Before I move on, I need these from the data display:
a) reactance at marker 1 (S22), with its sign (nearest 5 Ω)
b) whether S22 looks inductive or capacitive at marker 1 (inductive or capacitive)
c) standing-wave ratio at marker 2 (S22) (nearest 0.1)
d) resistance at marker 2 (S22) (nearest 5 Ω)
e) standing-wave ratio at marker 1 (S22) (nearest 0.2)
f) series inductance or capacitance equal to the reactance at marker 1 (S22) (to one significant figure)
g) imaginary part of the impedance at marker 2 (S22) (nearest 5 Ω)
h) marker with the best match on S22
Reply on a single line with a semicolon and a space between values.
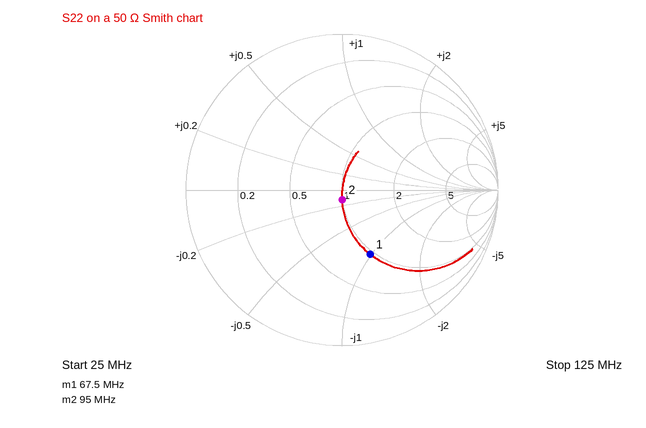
-50 Ω; capacitive; 1.1; 50 Ω; 2.6; 50 pF; -5 Ω; marker 2
